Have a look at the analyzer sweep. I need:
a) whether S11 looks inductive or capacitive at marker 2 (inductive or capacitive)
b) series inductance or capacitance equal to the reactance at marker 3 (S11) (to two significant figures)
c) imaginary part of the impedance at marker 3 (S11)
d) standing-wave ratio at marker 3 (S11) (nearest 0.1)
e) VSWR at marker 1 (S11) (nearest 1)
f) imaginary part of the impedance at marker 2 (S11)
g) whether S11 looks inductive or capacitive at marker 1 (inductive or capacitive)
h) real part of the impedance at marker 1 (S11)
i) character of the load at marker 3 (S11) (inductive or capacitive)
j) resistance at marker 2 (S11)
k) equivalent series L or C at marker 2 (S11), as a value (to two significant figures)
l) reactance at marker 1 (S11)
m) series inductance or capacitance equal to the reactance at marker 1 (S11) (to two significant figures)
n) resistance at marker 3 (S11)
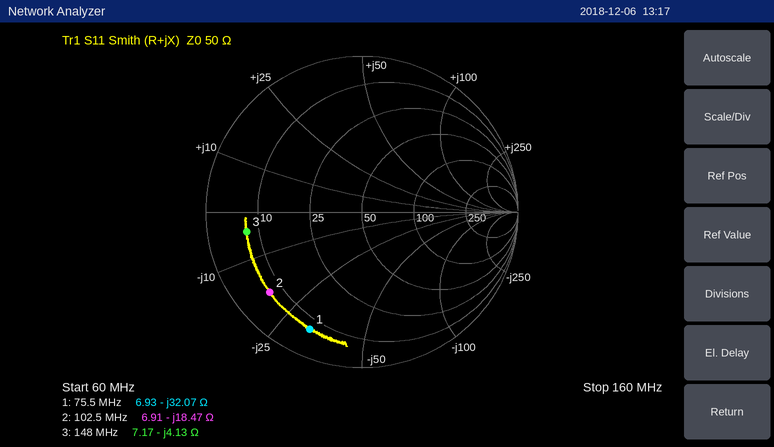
capacitive
260 pF
-4.13 Ω
7.0
10
-18.47 Ω
capacitive
6.93 Ω
capacitive
6.91 Ω
84 pF
-32.07 Ω
66 pF
7.17 Ω
